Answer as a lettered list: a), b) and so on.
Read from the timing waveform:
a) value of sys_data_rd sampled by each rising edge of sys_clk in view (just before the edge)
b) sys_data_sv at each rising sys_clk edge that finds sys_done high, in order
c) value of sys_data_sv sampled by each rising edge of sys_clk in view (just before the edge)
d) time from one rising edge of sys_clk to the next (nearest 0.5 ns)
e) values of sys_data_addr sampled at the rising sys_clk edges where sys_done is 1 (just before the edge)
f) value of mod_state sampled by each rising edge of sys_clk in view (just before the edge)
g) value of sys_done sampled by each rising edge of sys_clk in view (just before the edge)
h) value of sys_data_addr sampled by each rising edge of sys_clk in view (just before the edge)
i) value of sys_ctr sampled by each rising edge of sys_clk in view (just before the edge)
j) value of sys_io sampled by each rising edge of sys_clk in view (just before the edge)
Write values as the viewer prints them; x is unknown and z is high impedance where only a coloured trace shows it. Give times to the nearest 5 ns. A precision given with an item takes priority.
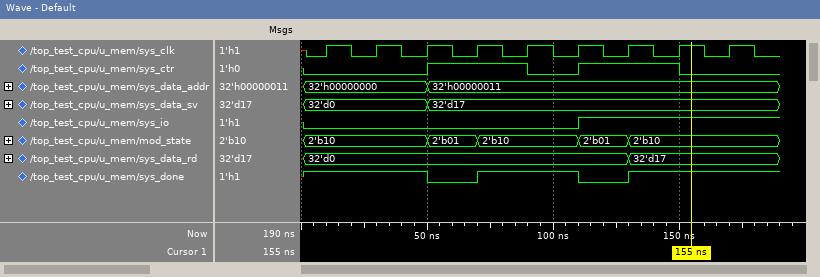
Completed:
a) 32'd0, 32'd0, 32'd0, 32'd0, 32'd0, 32'd0, 32'd0, 32'd17, 32'd17
b) 32'd0, 32'd0, 32'd0, 32'd17, 32'd17, 32'd17, 32'd17
c) 32'd0, 32'd0, 32'd0, 32'd17, 32'd17, 32'd17, 32'd17, 32'd17, 32'd17
d) 20 ns
e) 32'h00000000, 32'h00000000, 32'h00000000, 32'h00000011, 32'h00000011, 32'h00000011, 32'h00000011
f) 2'b10, 2'b10, 2'b10, 2'b01, 2'b10, 2'b10, 2'b01, 2'b10, 2'b10
g) 1 1 1 0 1 1 0 1 1
h) 32'h00000000, 32'h00000000, 32'h00000000, 32'h00000011, 32'h00000011, 32'h00000011, 32'h00000011, 32'h00000011, 32'h00000011
i) 0 0 0 1 1 0 1 1 0
j) 0 0 0 0 0 0 1 1 1
